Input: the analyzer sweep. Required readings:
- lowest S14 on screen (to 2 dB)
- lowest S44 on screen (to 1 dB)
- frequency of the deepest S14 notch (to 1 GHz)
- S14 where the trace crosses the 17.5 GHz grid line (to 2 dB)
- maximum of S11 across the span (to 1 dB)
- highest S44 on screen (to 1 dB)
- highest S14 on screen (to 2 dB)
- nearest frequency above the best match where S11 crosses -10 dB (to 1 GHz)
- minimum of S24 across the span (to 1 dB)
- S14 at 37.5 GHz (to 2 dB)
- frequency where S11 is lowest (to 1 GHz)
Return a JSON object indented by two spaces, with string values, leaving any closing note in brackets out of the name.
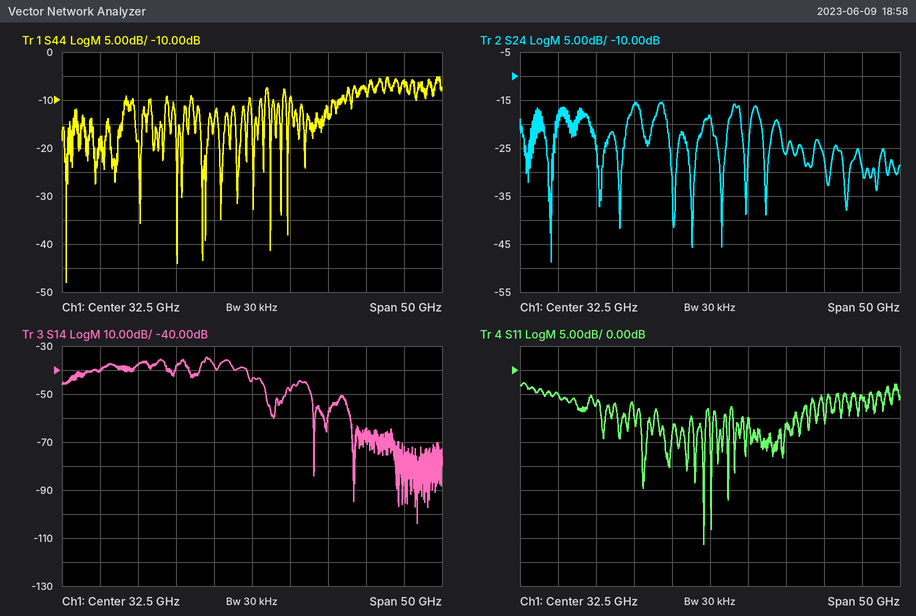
{
  "lowest S14 on screen": "-104 dB",
  "lowest S44 on screen": "-48 dB",
  "frequency of the deepest S14 notch": "54 GHz",
  "S14 where the trace crosses the 17.5 GHz grid line": "-38 dB",
  "maximum of S11 across the span": "-3 dB",
  "highest S44 on screen": "-5 dB",
  "highest S14 on screen": "-34 dB",
  "nearest frequency above the best match where S11 crosses -10 dB": "32 GHz",
  "minimum of S24 across the span": "-49 dB",
  "S14 at 37.5 GHz": "-48 dB",
  "frequency where S11 is lowest": "32 GHz"
}
